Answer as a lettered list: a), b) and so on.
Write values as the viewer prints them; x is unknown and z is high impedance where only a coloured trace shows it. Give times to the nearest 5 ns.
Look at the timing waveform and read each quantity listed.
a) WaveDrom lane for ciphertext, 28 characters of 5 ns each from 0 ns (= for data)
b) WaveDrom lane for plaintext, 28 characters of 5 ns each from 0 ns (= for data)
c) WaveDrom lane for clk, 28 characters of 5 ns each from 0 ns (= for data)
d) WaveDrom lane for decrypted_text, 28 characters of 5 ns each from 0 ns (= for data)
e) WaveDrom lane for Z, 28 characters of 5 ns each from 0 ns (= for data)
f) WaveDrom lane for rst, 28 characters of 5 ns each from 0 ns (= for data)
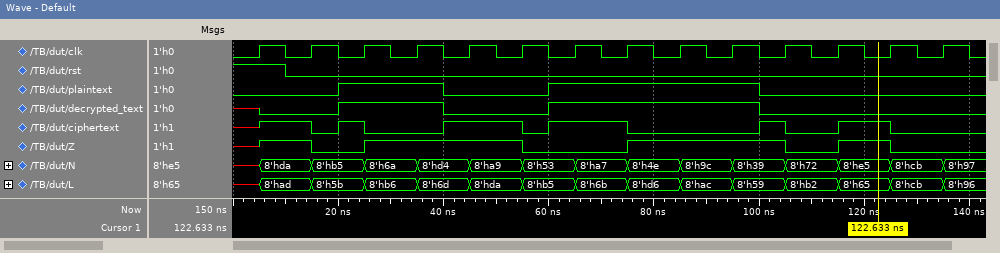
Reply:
a) {name: 'ciphertext', wave: 'x1.010..1..01..0....10.1.0..'}
b) {name: 'plaintext', wave: '0...1...0...1.......0.......'}
c) {name: 'clk', wave: '0101010101010101010101010101'}
d) {name: 'decrypted_text', wave: 'x0..1...0...1.......0.......'}
e) {name: 'Z', wave: 'x1.0.1.....0...1.....0.1.0..'}
f) {name: 'rst', wave: '1.0.........................'}
